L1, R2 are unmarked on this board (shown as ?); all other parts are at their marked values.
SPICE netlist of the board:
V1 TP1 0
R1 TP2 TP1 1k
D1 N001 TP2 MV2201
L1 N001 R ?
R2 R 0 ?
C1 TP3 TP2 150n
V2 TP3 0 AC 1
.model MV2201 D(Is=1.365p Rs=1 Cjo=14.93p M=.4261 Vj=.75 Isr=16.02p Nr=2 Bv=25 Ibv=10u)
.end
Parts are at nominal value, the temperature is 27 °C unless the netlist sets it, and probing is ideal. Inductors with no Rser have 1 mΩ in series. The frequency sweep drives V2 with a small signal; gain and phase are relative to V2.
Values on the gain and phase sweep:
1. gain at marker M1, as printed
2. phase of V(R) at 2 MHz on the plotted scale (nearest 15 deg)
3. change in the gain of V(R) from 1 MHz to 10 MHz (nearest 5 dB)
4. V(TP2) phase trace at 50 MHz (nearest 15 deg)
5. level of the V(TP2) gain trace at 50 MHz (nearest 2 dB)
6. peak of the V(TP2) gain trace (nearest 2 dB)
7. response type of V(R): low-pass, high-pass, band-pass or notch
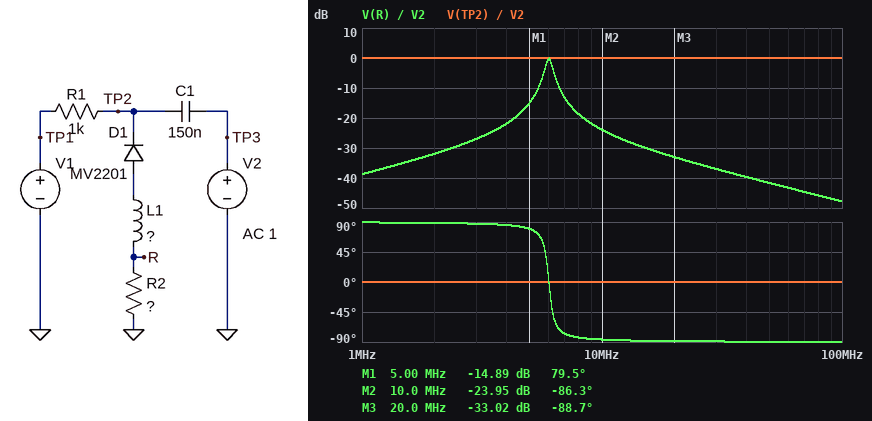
-14.89 dB
90 deg
15 dB
0 deg
0 dB
0 dB
band-pass
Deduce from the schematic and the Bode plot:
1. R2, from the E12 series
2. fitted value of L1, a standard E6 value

120 Ω
47 µH
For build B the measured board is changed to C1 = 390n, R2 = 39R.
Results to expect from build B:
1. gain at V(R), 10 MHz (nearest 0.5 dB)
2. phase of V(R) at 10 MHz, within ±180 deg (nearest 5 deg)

-33.5 dB
-90 deg
